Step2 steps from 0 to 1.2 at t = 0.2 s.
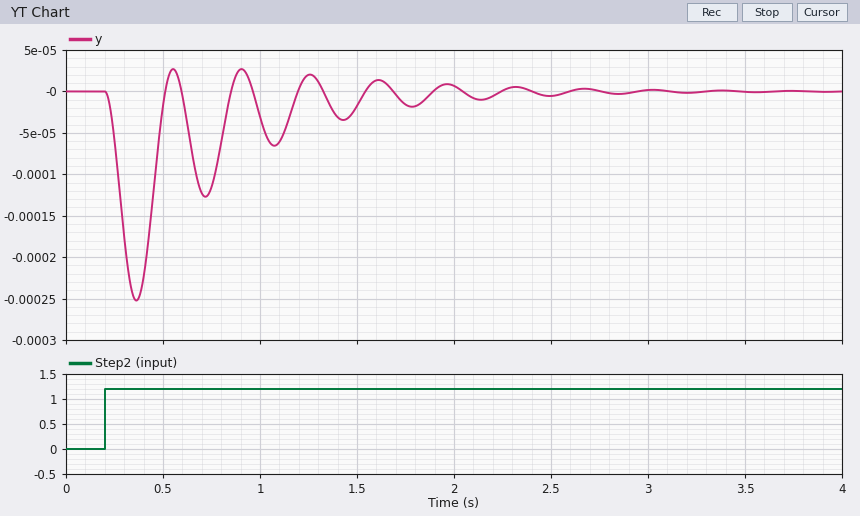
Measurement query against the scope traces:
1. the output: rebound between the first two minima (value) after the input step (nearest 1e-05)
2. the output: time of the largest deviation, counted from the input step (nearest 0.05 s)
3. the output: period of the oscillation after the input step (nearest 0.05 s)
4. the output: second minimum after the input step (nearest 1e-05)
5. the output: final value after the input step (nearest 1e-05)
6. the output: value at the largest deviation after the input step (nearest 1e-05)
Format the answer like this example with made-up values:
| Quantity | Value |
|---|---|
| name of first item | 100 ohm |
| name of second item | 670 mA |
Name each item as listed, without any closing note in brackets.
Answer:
| Quantity | Value |
|---|---|
| the output: rebound between the first two minima (value) after the input step | 0.00003 |
| the output: time of the largest deviation, counted from the input step | 0.15 s |
| the output: period of the oscillation after the input step | 0.35 s |
| the output: second minimum after the input step | -0.00013 |
| the output: final value after the input step | 0.00000 |
| the output: value at the largest deviation after the input step | -0.00025 |
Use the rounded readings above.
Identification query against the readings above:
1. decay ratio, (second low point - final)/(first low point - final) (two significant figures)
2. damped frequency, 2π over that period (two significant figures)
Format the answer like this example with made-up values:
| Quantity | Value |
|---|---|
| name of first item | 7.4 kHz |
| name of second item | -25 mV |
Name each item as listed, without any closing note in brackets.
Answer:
| Quantity | Value |
|---|---|
| decay ratio, (second low point - final)/(first low point - final) | 0.52 |
| damped frequency, 2π over that period | 18 rad/s |
